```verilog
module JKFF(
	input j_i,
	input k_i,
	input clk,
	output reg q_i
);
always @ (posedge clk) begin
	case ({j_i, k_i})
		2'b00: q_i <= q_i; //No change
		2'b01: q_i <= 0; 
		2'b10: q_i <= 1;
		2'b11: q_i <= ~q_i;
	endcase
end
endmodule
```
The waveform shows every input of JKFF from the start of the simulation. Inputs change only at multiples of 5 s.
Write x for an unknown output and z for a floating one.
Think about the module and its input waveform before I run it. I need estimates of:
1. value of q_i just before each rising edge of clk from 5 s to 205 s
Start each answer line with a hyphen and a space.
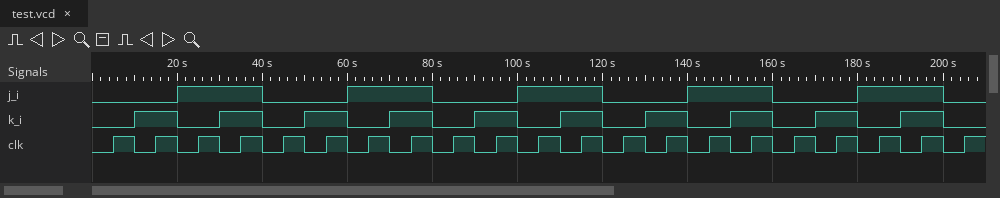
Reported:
- x x 0 1 0 0 0 1 0 0 0 1 0 0 0 1 0 0 0 1 0
